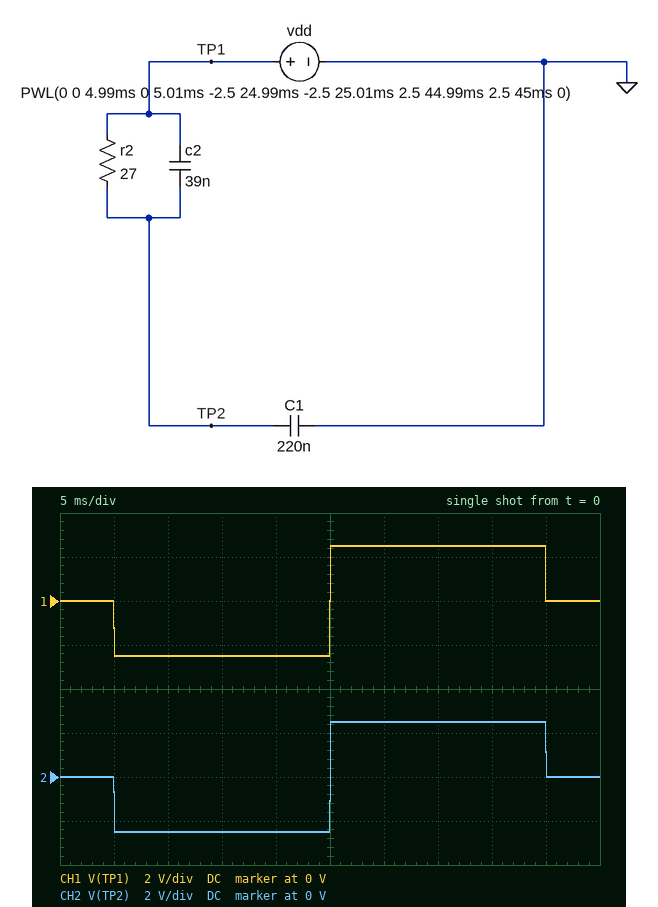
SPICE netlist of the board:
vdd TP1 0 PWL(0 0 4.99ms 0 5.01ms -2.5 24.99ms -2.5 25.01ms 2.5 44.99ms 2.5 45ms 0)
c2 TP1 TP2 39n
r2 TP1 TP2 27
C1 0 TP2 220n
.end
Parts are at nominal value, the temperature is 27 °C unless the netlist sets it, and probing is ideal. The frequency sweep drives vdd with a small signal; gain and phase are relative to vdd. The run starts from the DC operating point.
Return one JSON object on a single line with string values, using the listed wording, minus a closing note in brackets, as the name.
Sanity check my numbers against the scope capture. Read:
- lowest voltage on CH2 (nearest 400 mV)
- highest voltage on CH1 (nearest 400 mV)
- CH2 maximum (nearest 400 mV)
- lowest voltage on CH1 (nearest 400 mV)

{"lowest voltage on CH2": "-2.4 V", "highest voltage on CH1": "2.4 V", "CH2 maximum": "2.4 V", "lowest voltage on CH1": "-2.4 V"}
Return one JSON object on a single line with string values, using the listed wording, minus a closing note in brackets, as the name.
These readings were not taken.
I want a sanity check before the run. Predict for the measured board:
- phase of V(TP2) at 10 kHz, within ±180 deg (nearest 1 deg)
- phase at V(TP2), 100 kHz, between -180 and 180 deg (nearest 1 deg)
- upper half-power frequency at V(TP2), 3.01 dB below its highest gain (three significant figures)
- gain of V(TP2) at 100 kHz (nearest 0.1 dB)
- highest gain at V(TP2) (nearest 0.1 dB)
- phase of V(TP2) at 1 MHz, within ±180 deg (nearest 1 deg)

{"phase of V(TP2) at 10 kHz, within ±180 deg": "-20 deg", "phase at V(TP2), 100 kHz, between -180 and 180 deg": "-44 deg", "upper half-power frequency at V(TP2), 3.01 dB below its highest gain": "23.3 kHz", "gain of V(TP2) at 100 kHz": "-11.5 dB", "highest gain at V(TP2)": "0 dB", "phase of V(TP2) at 1 MHz, within ±180 deg": "-7 deg"}
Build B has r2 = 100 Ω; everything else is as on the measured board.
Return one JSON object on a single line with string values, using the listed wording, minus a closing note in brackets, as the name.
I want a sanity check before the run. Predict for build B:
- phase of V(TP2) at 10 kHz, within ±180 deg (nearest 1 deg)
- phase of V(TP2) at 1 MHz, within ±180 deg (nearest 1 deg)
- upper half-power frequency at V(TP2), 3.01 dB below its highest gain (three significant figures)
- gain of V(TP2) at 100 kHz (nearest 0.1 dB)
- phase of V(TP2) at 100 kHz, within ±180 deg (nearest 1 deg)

{"phase of V(TP2) at 10 kHz, within ±180 deg": "-45 deg", "phase of V(TP2) at 1 MHz, within ±180 deg": "-2 deg", "upper half-power frequency at V(TP2), 3.01 dB below its highest gain": "6.29 kHz", "gain of V(TP2) at 100 kHz": "-15.8 dB", "phase of V(TP2) at 100 kHz, within ±180 deg": "-19 deg"}
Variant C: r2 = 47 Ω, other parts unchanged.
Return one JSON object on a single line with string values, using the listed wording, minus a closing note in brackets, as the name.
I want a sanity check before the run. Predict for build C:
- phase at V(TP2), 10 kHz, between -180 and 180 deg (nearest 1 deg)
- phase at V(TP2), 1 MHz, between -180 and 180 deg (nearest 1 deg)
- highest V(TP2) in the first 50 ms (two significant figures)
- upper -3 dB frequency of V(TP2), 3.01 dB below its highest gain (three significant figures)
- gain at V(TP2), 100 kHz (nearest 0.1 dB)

{"phase at V(TP2), 10 kHz, between -180 and 180 deg": "-31 deg", "phase at V(TP2), 1 MHz, between -180 and 180 deg": "-4 deg", "highest V(TP2) in the first 50 ms": "2.5 V", "upper -3 dB frequency of V(TP2), 3.01 dB below its highest gain": "13.4 kHz", "gain at V(TP2), 100 kHz": "-14.1 dB"}
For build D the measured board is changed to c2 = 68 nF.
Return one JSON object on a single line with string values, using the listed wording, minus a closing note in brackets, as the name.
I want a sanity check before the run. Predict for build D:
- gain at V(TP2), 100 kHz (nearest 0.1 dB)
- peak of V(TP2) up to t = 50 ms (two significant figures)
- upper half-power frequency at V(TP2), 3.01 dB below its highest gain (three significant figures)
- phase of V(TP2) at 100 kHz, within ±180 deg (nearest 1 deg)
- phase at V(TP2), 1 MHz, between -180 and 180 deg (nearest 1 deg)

{"gain at V(TP2), 100 kHz": "-10.3 dB", "peak of V(TP2) up to t = 50 ms": "2.5 V", "upper half-power frequency at V(TP2), 3.01 dB below its highest gain": "21.7 kHz", "phase of V(TP2) at 100 kHz, within ±180 deg": "-29 deg", "phase at V(TP2), 1 MHz, between -180 and 180 deg": "-4 deg"}
